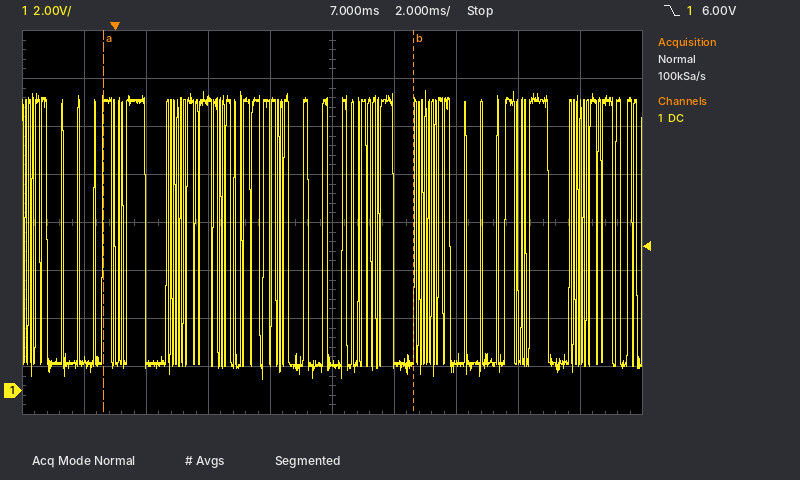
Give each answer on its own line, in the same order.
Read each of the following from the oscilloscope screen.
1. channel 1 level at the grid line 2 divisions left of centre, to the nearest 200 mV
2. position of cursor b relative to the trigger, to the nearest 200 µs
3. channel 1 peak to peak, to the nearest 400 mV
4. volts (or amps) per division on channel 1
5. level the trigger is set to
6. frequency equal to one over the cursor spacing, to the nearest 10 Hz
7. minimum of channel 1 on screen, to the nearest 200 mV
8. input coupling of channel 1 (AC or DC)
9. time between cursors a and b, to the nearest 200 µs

12.0 V
+9.6 ms
12.0 V
2 V
6.00 V
100 Hz
400 mV
DC
10.0 ms
